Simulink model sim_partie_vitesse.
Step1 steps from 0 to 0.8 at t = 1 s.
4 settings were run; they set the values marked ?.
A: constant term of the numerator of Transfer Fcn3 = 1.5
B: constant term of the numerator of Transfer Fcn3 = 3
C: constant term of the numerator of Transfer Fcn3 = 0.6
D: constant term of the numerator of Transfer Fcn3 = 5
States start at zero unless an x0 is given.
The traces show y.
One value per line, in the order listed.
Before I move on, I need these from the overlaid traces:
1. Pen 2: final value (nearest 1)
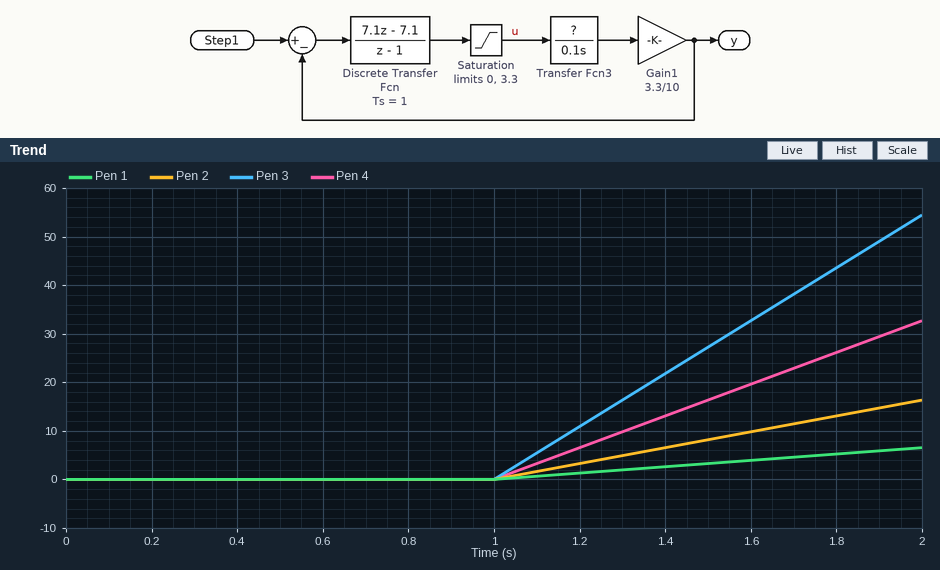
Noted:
16
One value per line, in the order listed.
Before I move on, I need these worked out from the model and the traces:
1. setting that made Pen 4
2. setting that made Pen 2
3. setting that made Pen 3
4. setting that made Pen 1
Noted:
B
A
D
C
